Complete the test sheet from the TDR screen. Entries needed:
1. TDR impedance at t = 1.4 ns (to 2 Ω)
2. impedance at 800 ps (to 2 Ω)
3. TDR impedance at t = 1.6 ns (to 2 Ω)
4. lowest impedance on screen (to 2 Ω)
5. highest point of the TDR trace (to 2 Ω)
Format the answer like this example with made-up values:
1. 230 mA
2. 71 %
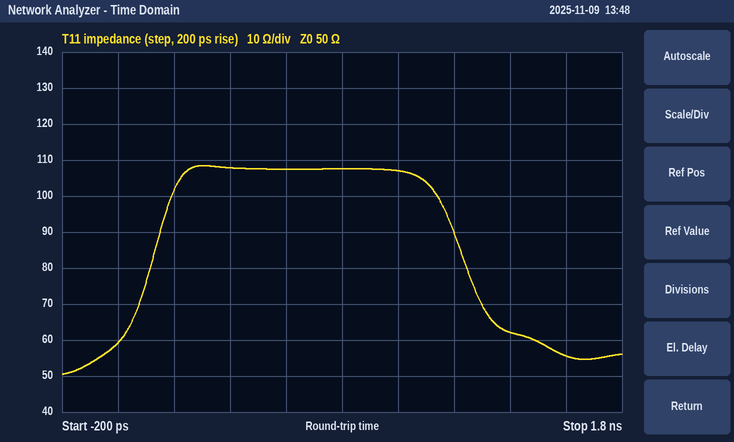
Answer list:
1. 62 Ω
2. 108 Ω
3. 56 Ω
4. 50 Ω
5. 108 Ω
